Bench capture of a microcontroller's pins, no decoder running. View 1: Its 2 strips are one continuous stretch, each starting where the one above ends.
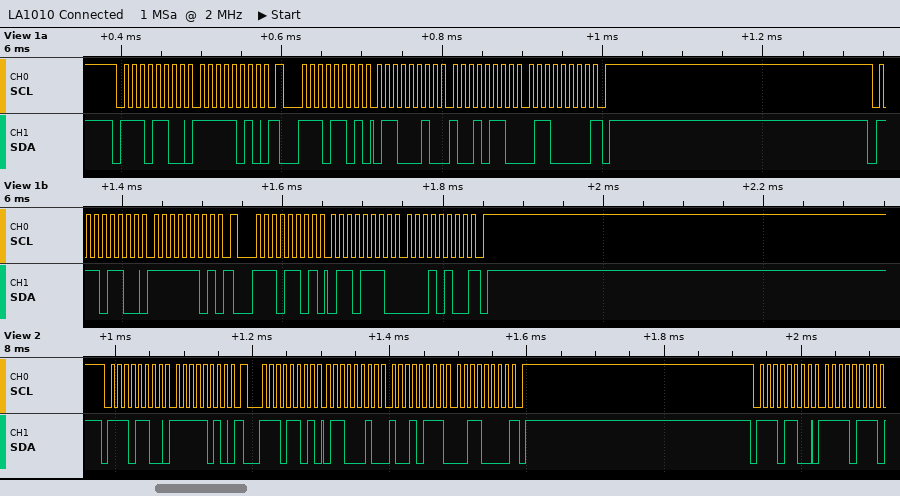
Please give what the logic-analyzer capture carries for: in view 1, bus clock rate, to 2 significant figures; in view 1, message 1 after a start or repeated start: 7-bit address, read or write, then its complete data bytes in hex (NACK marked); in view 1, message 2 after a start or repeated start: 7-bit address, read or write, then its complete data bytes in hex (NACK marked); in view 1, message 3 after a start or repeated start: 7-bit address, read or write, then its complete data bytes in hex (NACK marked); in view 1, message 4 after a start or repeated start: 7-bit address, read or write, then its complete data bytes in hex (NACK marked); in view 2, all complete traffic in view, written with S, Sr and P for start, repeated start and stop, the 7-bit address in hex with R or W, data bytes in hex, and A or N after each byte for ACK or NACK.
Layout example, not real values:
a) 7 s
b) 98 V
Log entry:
a) 100 kHz
b) 0x76 write: FA
c) 0x76 read: 62 96 60 NACK
d) 0x76 write: FD
e) 0x76 read: 6E 14 NACK
f) S 76W A FA A Sr 76R A 62 A 97 A 30 N P S 76W A F7 A
